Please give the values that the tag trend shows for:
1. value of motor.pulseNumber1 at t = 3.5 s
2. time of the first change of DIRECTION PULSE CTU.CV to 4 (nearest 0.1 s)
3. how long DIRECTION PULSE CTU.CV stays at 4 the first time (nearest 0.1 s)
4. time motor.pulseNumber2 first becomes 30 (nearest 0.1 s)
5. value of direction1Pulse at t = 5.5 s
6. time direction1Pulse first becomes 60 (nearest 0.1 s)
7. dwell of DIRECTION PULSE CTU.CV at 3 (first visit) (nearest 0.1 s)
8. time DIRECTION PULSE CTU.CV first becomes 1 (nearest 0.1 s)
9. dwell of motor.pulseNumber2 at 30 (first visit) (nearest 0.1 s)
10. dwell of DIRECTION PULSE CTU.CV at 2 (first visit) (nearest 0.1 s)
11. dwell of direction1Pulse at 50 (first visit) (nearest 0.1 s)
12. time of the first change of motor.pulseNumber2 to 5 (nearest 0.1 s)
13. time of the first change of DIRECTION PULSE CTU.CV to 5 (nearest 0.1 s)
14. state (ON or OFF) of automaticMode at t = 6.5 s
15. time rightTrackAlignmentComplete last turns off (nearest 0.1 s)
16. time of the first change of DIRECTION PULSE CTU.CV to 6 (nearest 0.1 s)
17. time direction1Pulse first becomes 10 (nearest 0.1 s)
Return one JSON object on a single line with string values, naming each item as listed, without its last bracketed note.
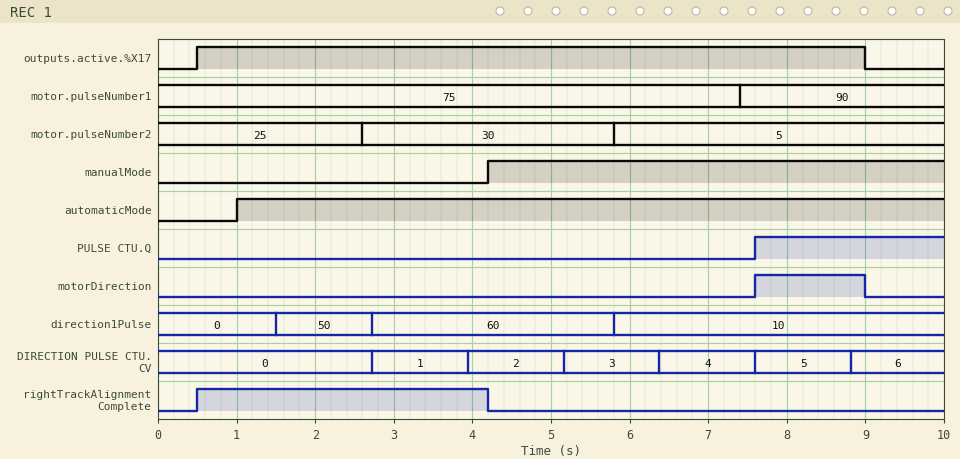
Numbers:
{"value of motor.pulseNumber1 at t = 3.5 s": "75", "time of the first change of DIRECTION PULSE CTU.CV to 4": "6.4 s", "how long DIRECTION PULSE CTU.CV stays at 4 the first time": "1.2 s", "time motor.pulseNumber2 first becomes 30": "2.6 s", "value of direction1Pulse at t = 5.5 s": "60", "time direction1Pulse first becomes 60": "2.7 s", "dwell of DIRECTION PULSE CTU.CV at 3 (first visit)": "1.2 s", "time DIRECTION PULSE CTU.CV first becomes 1": "2.7 s", "dwell of motor.pulseNumber2 at 30 (first visit)": "3.2 s", "dwell of DIRECTION PULSE CTU.CV at 2 (first visit)": "1.2 s", "dwell of direction1Pulse at 50 (first visit)": "1.2 s", "time of the first change of motor.pulseNumber2 to 5": "5.8 s", "time of the first change of DIRECTION PULSE CTU.CV to 5": "7.6 s", "state (ON or OFF) of automaticMode at t = 6.5 s": "ON", "time rightTrackAlignmentComplete last turns off": "4.2 s", "time of the first change of DIRECTION PULSE CTU.CV to 6": "8.8 s", "time direction1Pulse first becomes 10": "5.8 s"}
